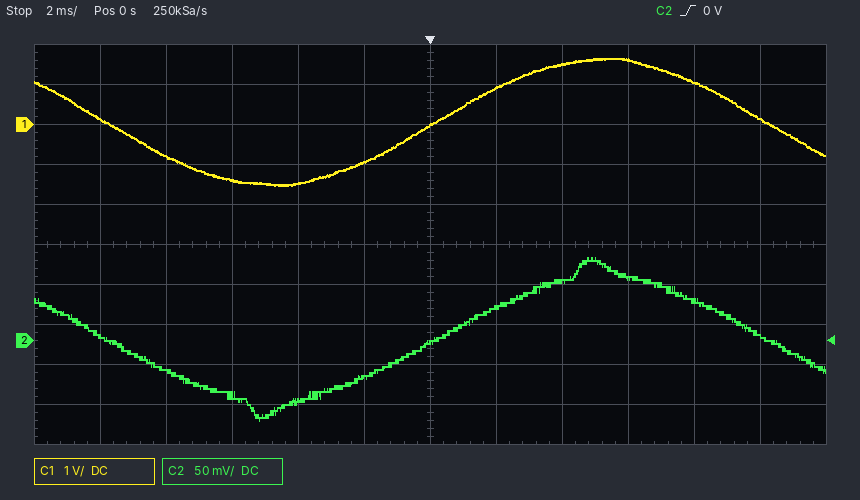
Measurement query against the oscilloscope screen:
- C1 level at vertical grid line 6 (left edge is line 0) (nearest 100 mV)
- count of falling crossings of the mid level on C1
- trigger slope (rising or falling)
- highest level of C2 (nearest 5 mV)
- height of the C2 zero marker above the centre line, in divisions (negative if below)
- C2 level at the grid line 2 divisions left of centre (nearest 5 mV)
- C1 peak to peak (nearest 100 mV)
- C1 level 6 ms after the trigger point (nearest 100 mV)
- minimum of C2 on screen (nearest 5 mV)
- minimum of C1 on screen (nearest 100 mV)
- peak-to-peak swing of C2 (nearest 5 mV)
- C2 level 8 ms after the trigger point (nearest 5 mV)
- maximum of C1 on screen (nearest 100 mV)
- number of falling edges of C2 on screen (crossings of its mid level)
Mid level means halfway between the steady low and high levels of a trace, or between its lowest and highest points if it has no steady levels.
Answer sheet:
0.0 V
2
rising
105 mV
-2.4 div
-75 mV
3.2 V
1.6 V
-100 mV
-1.5 V
205 mV
50 mV
1.7 V
2
